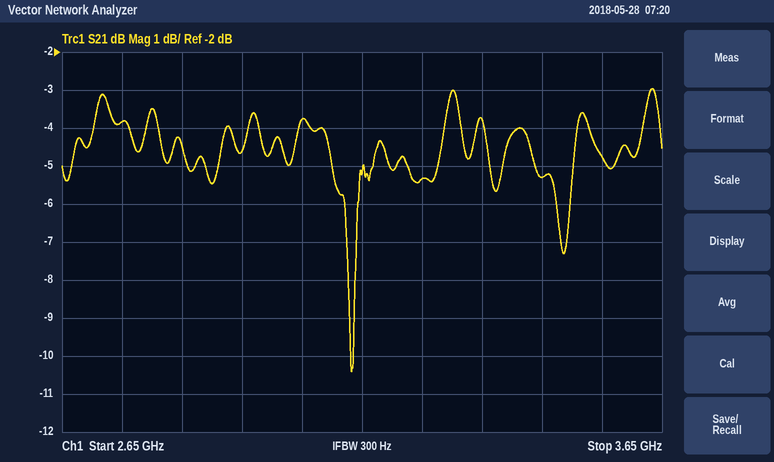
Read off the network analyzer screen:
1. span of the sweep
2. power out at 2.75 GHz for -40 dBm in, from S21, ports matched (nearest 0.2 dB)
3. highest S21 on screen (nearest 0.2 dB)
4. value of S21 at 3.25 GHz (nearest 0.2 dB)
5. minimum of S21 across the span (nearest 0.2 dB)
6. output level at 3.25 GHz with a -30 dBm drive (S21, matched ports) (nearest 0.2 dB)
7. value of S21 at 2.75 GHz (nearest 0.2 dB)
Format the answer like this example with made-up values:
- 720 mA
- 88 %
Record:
- 1 GHz
- -43.8 dBm
- -3.0 dB
- -5.4 dB
- -10.4 dB
- -35.4 dBm
- -3.8 dB
